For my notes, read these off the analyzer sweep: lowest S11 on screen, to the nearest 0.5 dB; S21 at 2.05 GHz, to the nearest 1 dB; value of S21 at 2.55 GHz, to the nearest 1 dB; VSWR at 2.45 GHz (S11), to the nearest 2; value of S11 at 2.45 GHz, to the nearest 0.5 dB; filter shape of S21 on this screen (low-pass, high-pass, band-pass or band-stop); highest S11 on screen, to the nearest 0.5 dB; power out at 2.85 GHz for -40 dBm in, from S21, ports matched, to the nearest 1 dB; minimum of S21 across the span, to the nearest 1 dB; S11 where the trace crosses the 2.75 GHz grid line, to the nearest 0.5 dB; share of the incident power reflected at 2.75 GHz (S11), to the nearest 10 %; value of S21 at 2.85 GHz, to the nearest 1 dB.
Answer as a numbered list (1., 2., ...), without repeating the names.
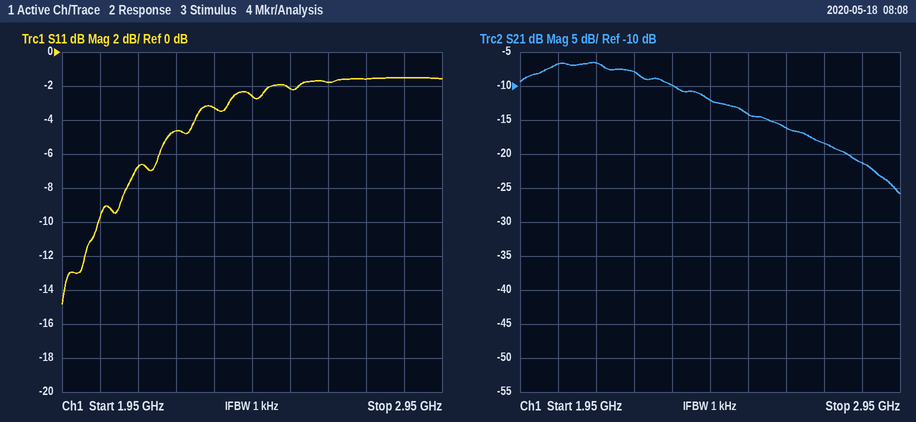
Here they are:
1. -15.0 dB
2. -7 dB
3. -14 dB
4. 6
5. -2.5 dB
6. low-pass
7. -1.5 dB
8. -61 dBm
9. -26 dB
10. -1.5 dB
11. 70 %
12. -21 dB
